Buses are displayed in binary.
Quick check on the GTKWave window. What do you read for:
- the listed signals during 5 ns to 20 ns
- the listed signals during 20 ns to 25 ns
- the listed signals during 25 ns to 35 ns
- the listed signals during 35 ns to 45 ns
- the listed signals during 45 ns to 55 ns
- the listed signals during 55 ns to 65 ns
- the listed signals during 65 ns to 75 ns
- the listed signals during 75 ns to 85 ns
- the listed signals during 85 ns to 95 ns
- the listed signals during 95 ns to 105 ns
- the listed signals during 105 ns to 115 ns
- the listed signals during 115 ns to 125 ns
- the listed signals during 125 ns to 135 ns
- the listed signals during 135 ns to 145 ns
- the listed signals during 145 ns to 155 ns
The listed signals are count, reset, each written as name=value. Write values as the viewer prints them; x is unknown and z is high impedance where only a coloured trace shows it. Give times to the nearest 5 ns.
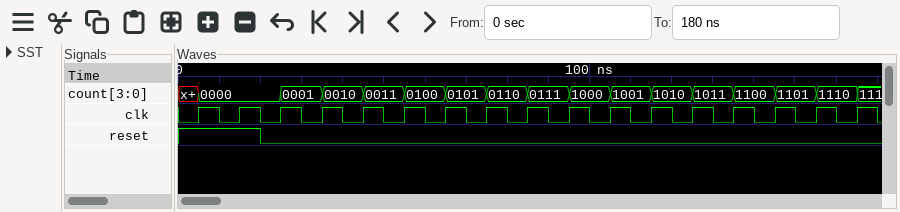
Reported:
count=0000, reset=1
count=0000, reset=0
count=0001, reset=0
count=0010, reset=0
count=0011, reset=0
count=0100, reset=0
count=0101, reset=0
count=0110, reset=0
count=0111, reset=0
count=1000, reset=0
count=1001, reset=0
count=1010, reset=0
count=1011, reset=0
count=1100, reset=0
count=1101, reset=0
